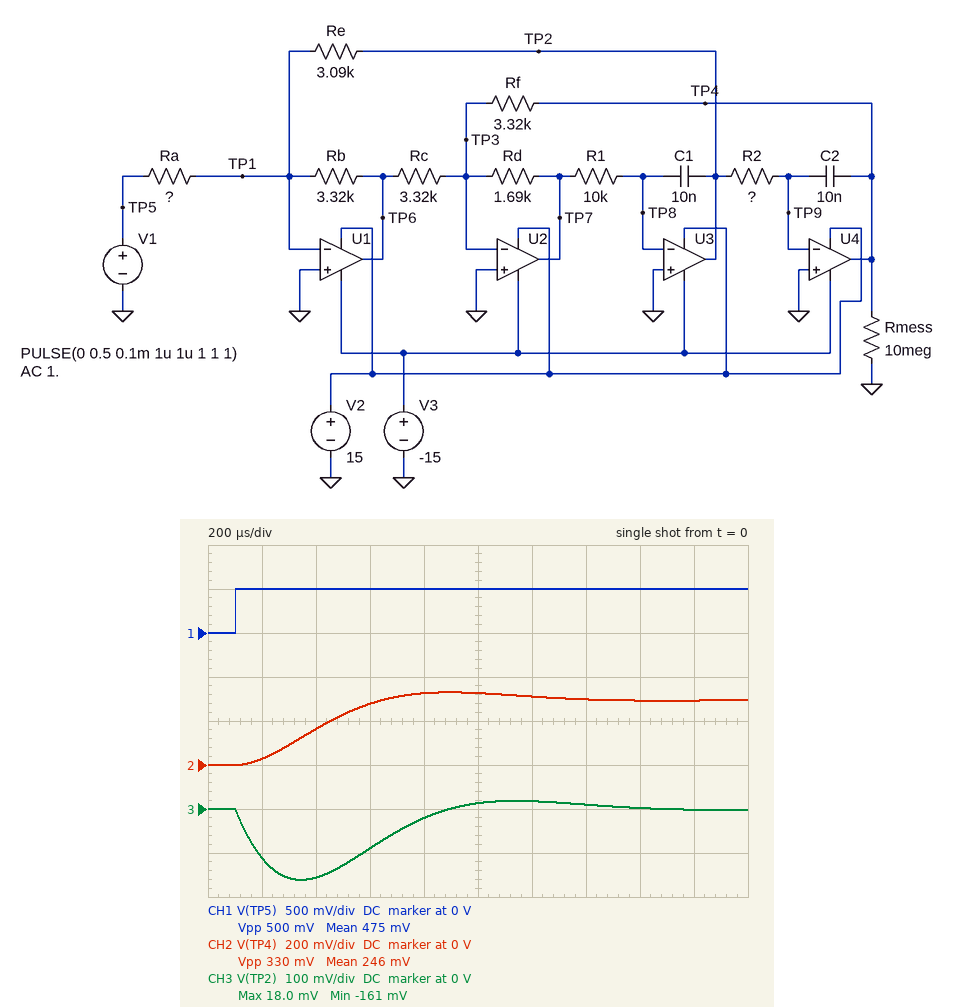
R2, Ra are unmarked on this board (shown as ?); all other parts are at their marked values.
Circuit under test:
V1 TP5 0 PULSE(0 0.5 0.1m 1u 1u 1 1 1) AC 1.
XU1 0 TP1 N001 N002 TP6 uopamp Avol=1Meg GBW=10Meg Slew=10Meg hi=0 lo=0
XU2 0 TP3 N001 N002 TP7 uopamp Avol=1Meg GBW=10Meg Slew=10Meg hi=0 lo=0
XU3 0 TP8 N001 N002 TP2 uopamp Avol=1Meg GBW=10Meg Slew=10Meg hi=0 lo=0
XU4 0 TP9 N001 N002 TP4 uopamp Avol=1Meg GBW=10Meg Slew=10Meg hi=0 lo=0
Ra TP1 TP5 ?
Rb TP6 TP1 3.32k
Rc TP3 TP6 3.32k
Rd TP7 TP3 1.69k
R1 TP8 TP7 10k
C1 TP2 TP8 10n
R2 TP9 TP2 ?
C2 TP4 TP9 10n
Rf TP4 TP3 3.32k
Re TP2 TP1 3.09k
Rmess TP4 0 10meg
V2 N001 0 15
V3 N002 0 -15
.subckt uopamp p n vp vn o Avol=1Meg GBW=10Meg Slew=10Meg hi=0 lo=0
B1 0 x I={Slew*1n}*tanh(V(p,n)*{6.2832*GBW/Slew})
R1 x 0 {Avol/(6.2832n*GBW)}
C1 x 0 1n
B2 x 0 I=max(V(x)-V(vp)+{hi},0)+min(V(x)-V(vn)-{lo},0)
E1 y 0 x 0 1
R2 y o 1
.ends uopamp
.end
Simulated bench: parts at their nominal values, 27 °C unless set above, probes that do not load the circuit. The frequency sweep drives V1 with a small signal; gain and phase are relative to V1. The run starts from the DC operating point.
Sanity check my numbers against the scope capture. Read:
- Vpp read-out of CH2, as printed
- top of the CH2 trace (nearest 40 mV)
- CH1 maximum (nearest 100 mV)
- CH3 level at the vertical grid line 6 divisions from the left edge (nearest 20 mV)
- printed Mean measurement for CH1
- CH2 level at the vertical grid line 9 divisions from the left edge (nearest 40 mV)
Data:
330 mV
320 mV
500 mV
20 mV
475 mV
280 mV
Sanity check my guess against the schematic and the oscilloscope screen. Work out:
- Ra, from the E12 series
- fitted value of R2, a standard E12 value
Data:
5.6 kΩ
22 kΩ
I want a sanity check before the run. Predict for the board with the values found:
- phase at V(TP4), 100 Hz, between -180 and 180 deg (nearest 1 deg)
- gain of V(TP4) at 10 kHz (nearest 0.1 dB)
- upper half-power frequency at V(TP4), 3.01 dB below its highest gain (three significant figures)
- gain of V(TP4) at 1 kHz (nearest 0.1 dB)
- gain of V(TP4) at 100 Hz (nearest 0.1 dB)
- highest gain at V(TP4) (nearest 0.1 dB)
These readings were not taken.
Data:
-9 deg
-49.2 dB
869 Hz
-8.9 dB
-4.5 dB
-4.0 dB
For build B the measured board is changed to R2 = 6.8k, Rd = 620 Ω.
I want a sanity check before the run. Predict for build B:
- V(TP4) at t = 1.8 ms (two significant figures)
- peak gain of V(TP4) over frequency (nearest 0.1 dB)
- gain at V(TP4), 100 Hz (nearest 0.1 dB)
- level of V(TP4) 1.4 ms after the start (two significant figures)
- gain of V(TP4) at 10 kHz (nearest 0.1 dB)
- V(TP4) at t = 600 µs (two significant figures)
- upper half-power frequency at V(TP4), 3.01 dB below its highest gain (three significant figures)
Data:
330 mV
4.0 dB
-4.4 dB
220 mV
-47.6 dB
430 mV
952 Hz
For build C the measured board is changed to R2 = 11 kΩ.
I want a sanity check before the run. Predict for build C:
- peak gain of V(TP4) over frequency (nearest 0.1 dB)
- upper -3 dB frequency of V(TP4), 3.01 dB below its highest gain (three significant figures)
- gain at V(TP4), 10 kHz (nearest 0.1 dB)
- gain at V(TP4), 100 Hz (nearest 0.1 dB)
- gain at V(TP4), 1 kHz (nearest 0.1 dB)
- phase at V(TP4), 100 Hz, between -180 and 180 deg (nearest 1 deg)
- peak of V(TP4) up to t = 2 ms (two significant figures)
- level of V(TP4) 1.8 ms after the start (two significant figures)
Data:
-1.9 dB
1.29 kHz
-43.1 dB
-4.5 dB
-2.1 dB
-4 deg
370 mV
300 mV
